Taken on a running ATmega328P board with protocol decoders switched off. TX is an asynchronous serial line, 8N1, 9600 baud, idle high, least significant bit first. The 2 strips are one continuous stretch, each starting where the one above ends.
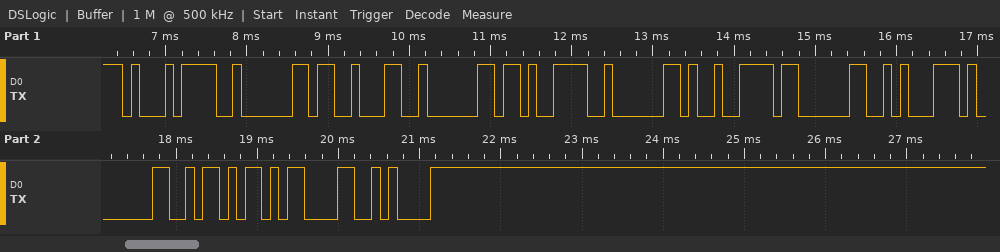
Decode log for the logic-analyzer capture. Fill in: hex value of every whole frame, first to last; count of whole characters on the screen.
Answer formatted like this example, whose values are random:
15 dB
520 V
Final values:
0xD1 0x02 0x13 0x02 0xCB 0x02 0xC9 0x03 0x8A 0x01 0x5A 0x0D 0x0A
13
